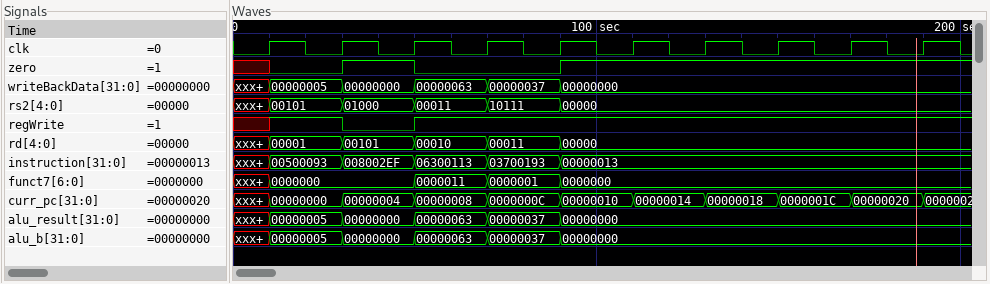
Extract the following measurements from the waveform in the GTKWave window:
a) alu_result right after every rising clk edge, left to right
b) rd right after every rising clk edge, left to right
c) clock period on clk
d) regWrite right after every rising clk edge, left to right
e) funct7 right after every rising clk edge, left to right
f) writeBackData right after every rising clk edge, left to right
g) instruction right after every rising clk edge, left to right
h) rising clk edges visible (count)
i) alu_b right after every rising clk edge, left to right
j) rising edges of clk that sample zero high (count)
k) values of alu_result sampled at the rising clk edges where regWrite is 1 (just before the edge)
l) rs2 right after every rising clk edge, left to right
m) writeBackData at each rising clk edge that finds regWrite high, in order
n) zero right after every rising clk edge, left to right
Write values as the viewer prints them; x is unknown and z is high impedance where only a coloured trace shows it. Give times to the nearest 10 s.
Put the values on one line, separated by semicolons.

00000005, 00000000, 00000063, 00000037, 00000000, 00000000, 00000000, 00000000, 00000000, 00000000; 00001, 00101, 00010, 00011, 00000, 00000, 00000, 00000, 00000, 00000; 20 s; 1 0 1 1 1 1 1 1 1 1; 0000000, 0000000, 0000011, 0000001, 0000000, 0000000, 0000000, 0000000, 0000000, 0000000; 00000005, 00000000, 00000063, 00000037, 00000000, 00000000, 00000000, 00000000, 00000000, 00000000; 00500093, 008002EF, 06300113, 03700193, 00000013, 00000013, 00000013, 00000013, 00000013, 00000013; 10; 00000005, 00000000, 00000063, 00000037, 00000000, 00000000, 00000000, 00000000, 00000000, 00000000; 6; 00000005, 00000063, 00000037, 00000000, 00000000, 00000000, 00000000, 00000000; 00101, 01000, 00011, 10111, 00000, 00000, 00000, 00000, 00000, 00000; 00000005, 00000063, 00000037, 00000000, 00000000, 00000000, 00000000, 00000000; 0 1 0 0 1 1 1 1 1 1
